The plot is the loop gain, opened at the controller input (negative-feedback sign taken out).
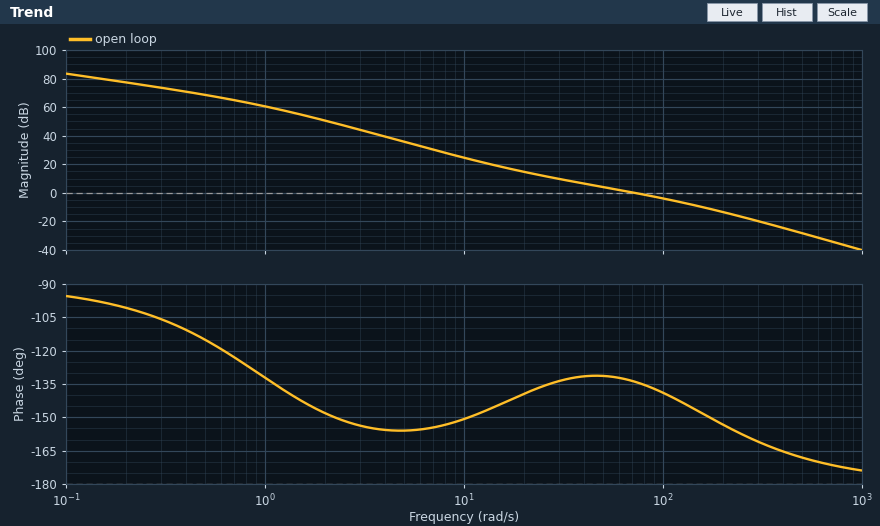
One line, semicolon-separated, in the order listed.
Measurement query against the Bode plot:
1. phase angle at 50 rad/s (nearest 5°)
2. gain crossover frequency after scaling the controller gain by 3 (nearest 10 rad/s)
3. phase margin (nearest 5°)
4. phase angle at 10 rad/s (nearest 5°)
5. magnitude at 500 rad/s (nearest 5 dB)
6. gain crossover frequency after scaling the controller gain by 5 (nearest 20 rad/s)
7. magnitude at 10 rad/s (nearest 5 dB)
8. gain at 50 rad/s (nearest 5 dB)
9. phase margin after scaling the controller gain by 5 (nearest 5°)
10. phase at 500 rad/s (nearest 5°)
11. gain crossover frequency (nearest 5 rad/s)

-130°; 150 rad/s; 45°; -150°; -30 dB; 200 rad/s; 25 dB; 5 dB; 25°; -170°; 70 rad/s
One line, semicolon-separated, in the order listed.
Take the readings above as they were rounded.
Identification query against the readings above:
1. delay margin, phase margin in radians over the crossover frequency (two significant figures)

0.011 s
